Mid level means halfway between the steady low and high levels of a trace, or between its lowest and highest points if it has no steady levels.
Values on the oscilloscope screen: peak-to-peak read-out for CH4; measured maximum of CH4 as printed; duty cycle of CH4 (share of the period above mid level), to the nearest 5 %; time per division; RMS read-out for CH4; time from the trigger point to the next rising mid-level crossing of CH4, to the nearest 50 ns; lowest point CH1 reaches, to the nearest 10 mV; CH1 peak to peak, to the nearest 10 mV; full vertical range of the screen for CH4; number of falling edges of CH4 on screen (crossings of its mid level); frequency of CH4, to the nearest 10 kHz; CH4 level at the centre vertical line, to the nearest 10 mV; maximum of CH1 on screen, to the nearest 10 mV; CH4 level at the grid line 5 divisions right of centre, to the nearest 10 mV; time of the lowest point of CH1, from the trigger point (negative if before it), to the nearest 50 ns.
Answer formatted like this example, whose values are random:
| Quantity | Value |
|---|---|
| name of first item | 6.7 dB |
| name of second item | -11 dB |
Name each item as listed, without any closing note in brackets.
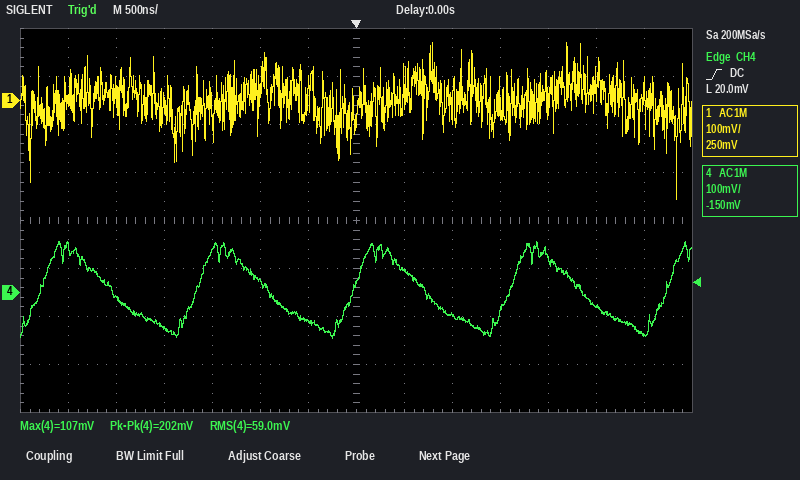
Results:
| Quantity | Value |
|---|---|
| peak-to-peak read-out for CH4 | 202 mV |
| measured maximum of CH4 as printed | 107 mV |
| duty cycle of CH4 (share of the period above mid level), to the nearest 5 % | 45 % |
| time per division | 500 ns |
| RMS read-out for CH4 | 59.0 mV |
| time from the trigger point to the next rising mid-level crossing of CH4, to the nearest 50 ns | 1.60 µs |
| lowest point CH1 reaches, to the nearest 10 mV | -210 mV |
| CH1 peak to peak, to the nearest 10 mV | 330 mV |
| full vertical range of the screen for CH4 | 800 mV |
| number of falling edges of CH4 on screen | 4 |
| frequency of CH4, to the nearest 10 kHz | 610 kHz |
| CH4 level at the centre vertical line, to the nearest 10 mV | 20 mV |
| maximum of CH1 on screen, to the nearest 10 mV | 120 mV |
| CH4 level at the grid line 5 divisions right of centre, to the nearest 10 mV | -30 mV |
| time of the lowest point of CH1, from the trigger point (negative if before it), to the nearest 50 ns | +3.35 µs |
